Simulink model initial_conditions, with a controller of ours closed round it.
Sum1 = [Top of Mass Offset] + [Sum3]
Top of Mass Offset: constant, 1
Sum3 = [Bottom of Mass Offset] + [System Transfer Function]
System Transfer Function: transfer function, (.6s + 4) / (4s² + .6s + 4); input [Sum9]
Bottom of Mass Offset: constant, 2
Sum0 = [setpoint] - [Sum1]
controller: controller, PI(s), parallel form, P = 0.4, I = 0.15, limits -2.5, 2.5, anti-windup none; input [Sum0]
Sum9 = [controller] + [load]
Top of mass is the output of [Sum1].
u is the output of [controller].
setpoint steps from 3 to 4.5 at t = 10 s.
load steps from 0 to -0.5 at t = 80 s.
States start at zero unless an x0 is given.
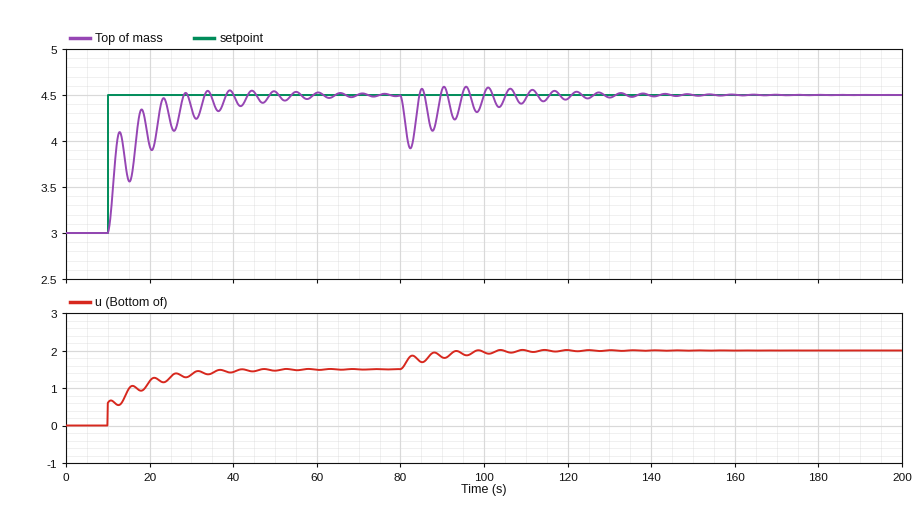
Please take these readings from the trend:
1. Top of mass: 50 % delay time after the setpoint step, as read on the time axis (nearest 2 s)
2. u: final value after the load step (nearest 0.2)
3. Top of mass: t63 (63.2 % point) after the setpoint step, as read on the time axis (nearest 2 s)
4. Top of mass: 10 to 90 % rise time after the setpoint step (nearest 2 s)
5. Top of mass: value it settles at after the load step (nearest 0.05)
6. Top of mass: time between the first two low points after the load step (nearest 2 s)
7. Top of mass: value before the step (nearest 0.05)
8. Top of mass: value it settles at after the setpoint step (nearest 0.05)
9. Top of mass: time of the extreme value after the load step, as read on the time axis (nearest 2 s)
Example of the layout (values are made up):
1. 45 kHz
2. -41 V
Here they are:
1. 12 s
2. 2.0
3. 12 s
4. 12 s
5. 4.50
6. 6 s
7. 3.00
8. 4.50
9. 82 s
